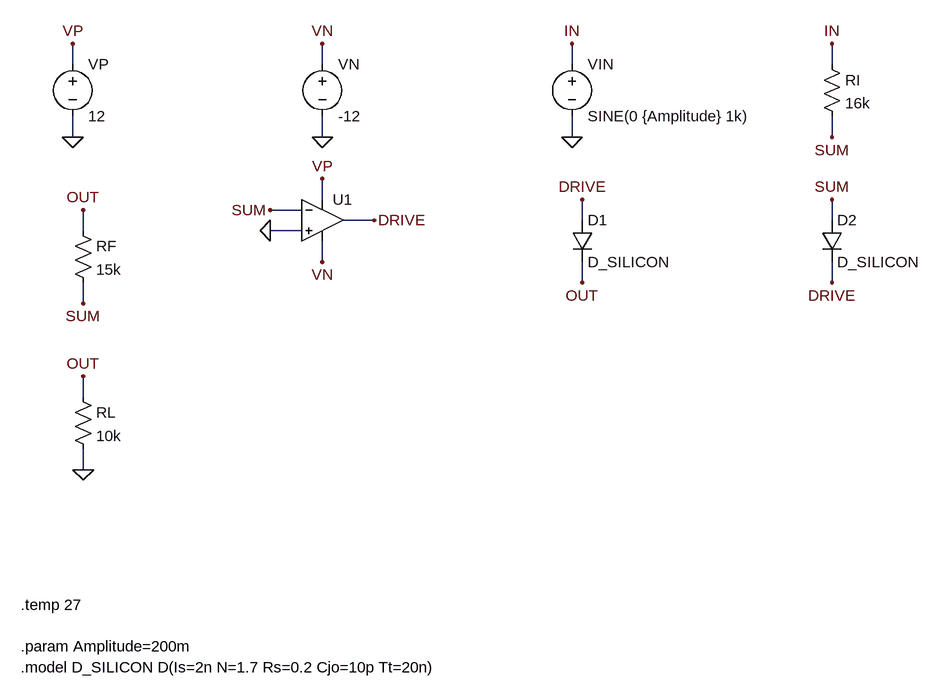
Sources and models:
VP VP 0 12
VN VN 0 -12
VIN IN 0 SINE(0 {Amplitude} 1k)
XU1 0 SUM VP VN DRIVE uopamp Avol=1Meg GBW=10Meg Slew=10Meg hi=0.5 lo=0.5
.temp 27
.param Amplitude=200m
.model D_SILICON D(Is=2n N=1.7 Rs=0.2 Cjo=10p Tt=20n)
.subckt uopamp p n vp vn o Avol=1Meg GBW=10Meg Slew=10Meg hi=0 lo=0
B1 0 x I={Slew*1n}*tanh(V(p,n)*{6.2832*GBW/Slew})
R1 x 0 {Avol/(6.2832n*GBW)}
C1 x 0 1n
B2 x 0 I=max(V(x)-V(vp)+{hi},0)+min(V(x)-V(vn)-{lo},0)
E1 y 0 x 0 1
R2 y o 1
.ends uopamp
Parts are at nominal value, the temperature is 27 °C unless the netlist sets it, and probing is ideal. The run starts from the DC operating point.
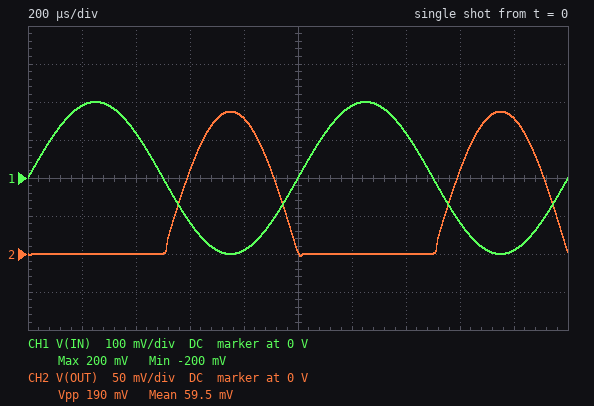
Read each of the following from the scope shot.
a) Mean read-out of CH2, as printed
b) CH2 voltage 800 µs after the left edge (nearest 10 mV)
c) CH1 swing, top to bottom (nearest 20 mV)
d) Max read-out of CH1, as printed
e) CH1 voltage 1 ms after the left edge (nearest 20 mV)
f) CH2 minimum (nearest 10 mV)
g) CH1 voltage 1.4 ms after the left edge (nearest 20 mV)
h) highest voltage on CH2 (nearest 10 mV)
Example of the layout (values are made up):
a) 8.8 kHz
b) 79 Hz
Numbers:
a) 59.5 mV
b) 180 mV
c) 400 mV
d) 200 mV
e) 0 V
f) 0 V
g) 120 mV
h) 190 mV
